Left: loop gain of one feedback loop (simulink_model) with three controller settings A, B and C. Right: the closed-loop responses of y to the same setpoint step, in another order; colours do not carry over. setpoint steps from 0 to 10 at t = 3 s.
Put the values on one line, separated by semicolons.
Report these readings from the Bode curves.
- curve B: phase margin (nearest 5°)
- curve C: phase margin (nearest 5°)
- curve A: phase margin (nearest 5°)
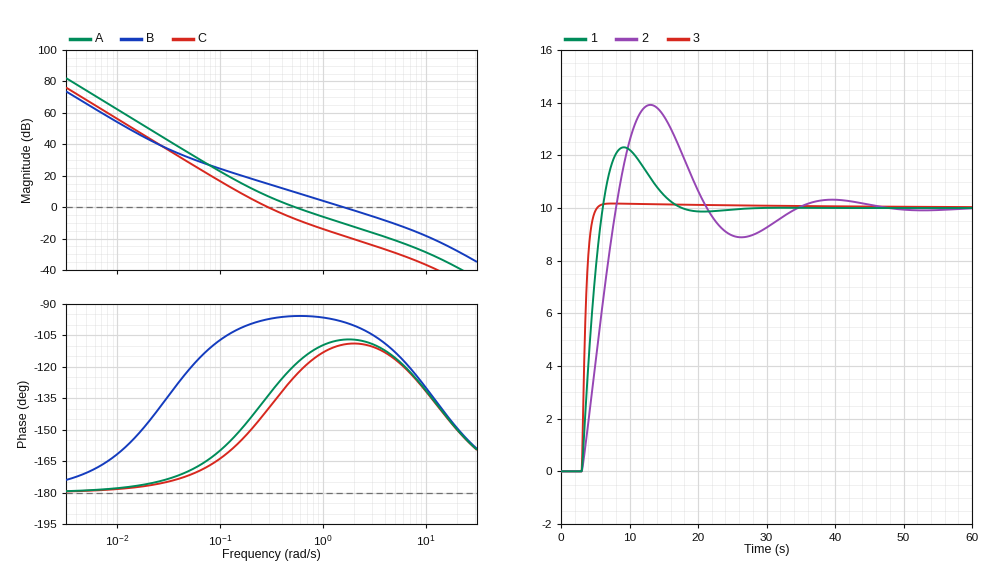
80°; 40°; 60°
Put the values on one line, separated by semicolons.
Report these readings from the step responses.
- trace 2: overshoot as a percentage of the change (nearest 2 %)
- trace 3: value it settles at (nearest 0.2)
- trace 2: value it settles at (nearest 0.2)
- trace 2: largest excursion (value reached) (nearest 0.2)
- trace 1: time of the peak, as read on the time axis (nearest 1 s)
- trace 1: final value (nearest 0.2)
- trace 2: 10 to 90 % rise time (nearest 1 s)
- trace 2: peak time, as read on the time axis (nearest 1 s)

40 %; 10.0; 10.0; 14.0; 9 s; 10.0; 4 s; 13 s
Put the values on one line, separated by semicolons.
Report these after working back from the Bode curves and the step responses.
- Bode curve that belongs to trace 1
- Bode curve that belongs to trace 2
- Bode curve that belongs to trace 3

A; C; B
